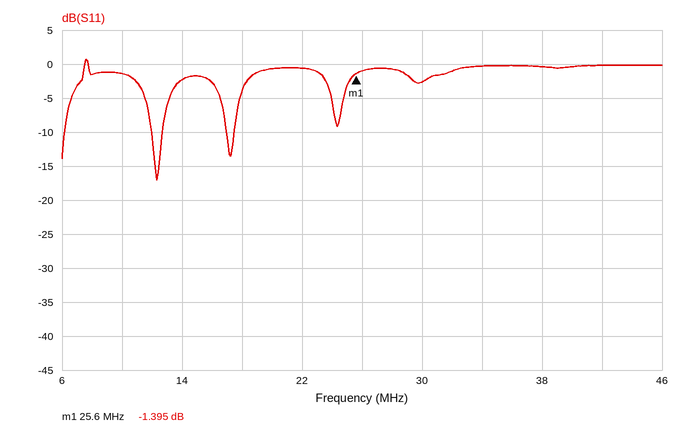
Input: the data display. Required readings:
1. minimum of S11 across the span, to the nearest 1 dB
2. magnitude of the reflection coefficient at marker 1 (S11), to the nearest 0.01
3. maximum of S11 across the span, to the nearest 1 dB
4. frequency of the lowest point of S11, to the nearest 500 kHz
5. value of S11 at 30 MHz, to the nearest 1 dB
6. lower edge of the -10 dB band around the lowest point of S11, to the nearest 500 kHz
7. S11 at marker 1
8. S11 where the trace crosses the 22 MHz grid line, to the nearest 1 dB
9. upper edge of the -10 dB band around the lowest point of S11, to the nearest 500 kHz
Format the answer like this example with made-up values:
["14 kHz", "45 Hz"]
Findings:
["-17 dB", "0.85", "1 dB", "12.5 MHz", "-3 dB", "12.0 MHz", "-1.395 dB", "-1 dB", "12.5 MHz"]
